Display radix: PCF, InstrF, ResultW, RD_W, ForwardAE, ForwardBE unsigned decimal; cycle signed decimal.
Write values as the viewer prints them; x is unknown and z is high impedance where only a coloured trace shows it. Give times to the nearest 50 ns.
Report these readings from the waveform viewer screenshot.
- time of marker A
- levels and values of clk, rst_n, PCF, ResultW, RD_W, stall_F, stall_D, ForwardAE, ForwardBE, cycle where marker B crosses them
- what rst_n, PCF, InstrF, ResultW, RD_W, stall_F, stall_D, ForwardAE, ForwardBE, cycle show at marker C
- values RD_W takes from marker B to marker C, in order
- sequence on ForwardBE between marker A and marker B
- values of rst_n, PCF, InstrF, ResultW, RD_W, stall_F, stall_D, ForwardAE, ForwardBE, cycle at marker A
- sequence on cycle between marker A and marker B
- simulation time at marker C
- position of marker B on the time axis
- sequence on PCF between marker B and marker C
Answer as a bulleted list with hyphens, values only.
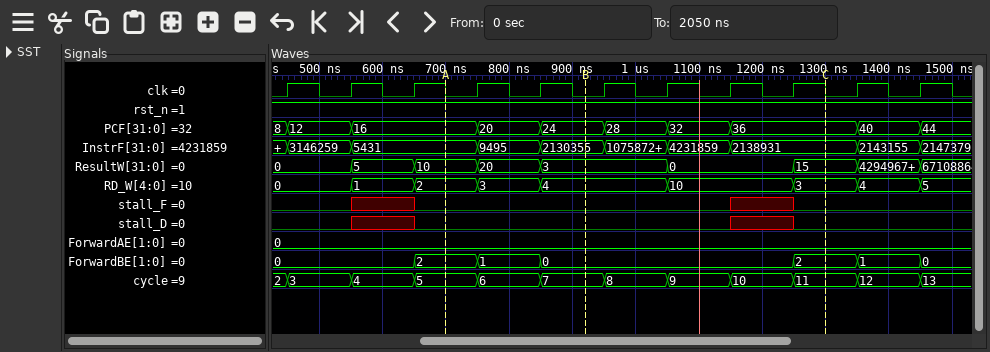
- 700 ns
- clk=0, rst_n=1, PCF=24, ResultW=3, RD_W=4, stall_F=0, stall_D=0, ForwardAE=0, ForwardBE=0, cycle=7
- rst_n=1, PCF=36, InstrF=2138931, ResultW=15, RD_W=3, stall_F=0, stall_D=0, ForwardAE=0, ForwardBE=2, cycle=11
- 4, 10, 3
- 2, 1, 0
- rst_n=1, PCF=16, InstrF=5431, ResultW=10, RD_W=2, stall_F=0, stall_D=0, ForwardAE=0, ForwardBE=2, cycle=5
- 5, 6, 7
- 1300 ns
- 900 ns
- 24, 28, 32, 36
